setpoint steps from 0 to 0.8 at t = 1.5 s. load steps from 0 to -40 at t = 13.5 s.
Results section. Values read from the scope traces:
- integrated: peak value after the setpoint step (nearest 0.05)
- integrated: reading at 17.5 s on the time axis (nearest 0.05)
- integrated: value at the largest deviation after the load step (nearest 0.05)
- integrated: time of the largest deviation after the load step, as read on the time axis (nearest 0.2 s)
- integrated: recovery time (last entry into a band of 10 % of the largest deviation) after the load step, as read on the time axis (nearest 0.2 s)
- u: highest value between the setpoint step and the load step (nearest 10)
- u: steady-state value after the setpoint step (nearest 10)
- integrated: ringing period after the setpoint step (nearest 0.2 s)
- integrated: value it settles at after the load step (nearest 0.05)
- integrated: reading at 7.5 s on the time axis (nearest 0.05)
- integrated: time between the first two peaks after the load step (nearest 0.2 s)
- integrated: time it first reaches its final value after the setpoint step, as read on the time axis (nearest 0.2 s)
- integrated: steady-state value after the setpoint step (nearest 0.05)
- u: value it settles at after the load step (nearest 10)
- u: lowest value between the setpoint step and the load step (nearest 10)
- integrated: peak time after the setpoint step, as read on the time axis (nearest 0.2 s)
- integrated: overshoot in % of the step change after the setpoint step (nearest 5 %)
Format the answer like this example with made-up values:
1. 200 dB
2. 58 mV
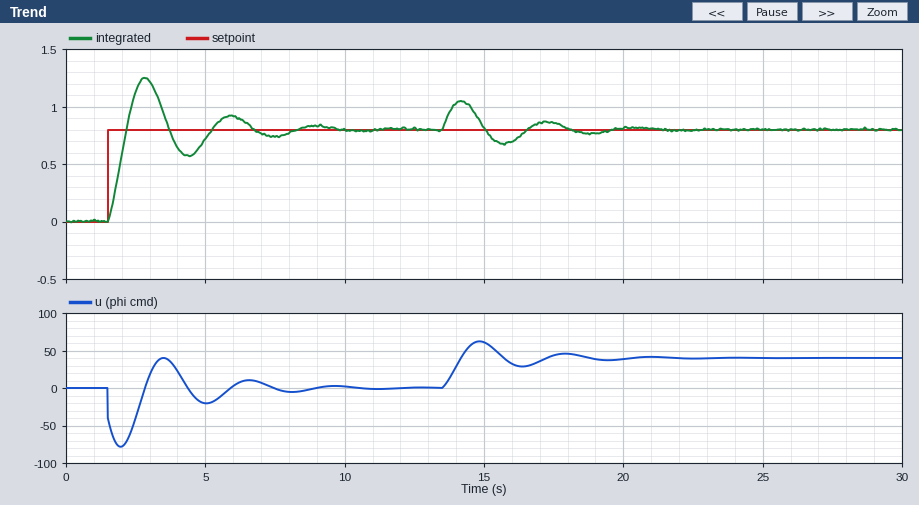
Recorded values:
1. 1.25
2. 0.85
3. 1.05
4. 14.2 s
5. 19.2 s
6. 40
7. 0
8. 3.0 s
9. 0.80
10. 0.75
11. 3.0 s
12. 2.2 s
13. 0.80
14. 40
15. -80
16. 2.8 s
17. 55 %
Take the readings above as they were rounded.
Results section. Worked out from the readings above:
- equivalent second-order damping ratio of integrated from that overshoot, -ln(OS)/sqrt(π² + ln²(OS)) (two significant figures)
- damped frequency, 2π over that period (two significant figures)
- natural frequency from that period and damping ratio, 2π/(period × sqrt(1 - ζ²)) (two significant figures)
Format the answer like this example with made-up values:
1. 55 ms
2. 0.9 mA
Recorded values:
1. 0.19
2. 2.1 rad/s
3. 2.1 rad/s
